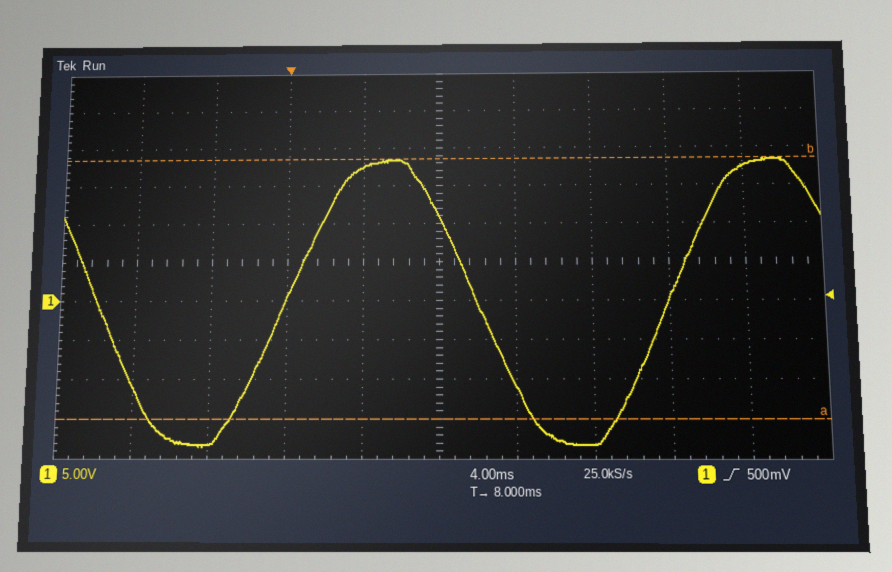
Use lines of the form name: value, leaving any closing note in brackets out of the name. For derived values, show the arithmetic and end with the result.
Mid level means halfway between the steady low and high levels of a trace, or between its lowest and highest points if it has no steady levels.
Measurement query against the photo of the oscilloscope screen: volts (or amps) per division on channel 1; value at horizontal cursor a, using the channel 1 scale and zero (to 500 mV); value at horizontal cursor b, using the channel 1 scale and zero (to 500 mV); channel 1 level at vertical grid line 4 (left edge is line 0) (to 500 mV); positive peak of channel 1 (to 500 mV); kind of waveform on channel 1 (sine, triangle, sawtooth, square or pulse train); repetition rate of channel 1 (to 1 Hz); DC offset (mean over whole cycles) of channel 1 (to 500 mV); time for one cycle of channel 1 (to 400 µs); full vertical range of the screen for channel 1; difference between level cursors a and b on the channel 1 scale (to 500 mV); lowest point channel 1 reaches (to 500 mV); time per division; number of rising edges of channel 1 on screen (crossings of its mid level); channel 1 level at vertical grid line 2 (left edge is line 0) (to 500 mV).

volts (or amps) per division on channel 1: 5 V
value at horizontal cursor a, using the channel 1 scale and zero: -15.0 V
value at horizontal cursor b, using the channel 1 scale and zero: 18.5 V
channel 1 level at vertical grid line 4 (left edge is line 0): 17.5 V
positive peak of channel 1: 18.5 V
kind of waveform on channel 1: sine
repetition rate of channel 1: 1 / 20.0 ms ≈ 50 Hz
DC offset (mean over whole cycles) of channel 1: (18.5 V + (-18.5 V)) / 2 ≈ 0.0 V
time for one cycle of channel 1: 20.0 ms
full vertical range of the screen for channel 1: 50 V
difference between level cursors a and b on the channel 1 scale: 33.5 V
lowest point channel 1 reaches: -18.5 V
time per division: 4 ms
number of rising edges of channel 1 on screen: 2
channel 1 level at vertical grid line 2 (left edge is line 0): -18.0 V
